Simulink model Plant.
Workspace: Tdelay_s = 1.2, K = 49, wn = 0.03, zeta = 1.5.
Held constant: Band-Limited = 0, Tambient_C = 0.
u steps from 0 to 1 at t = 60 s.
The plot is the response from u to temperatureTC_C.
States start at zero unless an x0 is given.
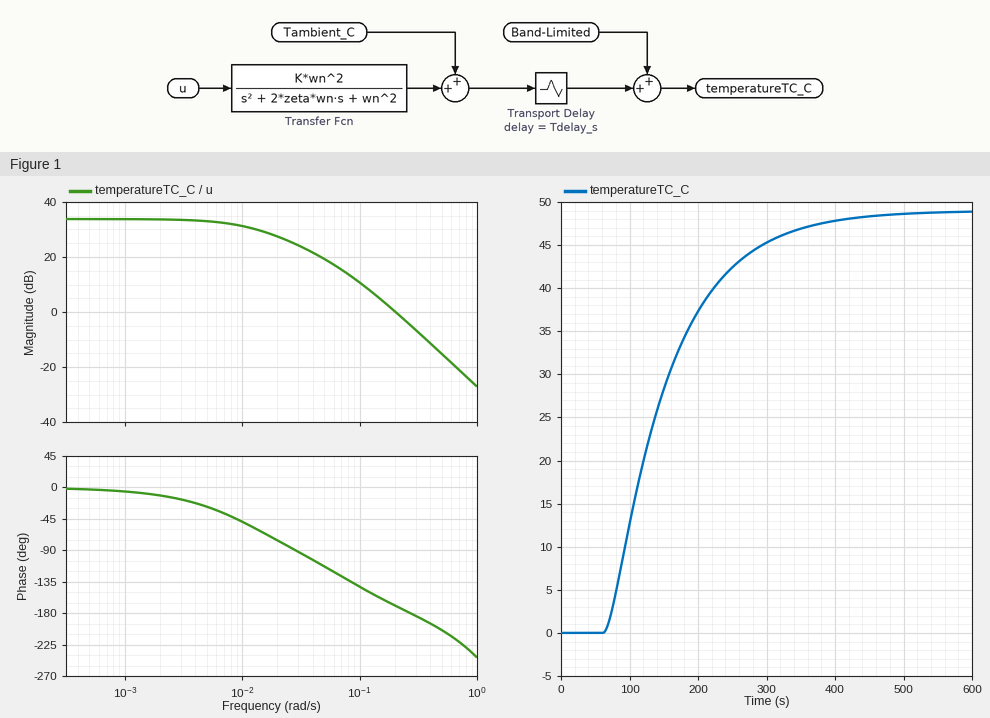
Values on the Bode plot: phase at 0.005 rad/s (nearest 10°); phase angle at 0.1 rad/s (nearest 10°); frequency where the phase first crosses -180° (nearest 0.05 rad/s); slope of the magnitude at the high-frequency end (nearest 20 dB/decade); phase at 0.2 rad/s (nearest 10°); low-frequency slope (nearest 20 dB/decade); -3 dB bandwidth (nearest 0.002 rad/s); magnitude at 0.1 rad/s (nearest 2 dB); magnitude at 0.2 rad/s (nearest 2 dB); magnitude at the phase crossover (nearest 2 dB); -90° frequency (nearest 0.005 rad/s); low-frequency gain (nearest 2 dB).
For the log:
-30°
-140°
0.25 rad/s
-40 dB/decade
-170°
0 dB/decade
0.012 rad/s
10 dB
0 dB
-4 dB
0.030 rad/s
34 dB
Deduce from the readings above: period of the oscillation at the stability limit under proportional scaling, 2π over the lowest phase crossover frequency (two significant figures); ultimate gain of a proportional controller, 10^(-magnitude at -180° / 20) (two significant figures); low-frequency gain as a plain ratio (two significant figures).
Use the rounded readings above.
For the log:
25 s
1.6
50
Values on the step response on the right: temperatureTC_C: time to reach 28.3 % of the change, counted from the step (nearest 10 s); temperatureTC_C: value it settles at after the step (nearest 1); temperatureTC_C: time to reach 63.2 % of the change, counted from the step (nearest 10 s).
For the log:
40 s
49
100 s
